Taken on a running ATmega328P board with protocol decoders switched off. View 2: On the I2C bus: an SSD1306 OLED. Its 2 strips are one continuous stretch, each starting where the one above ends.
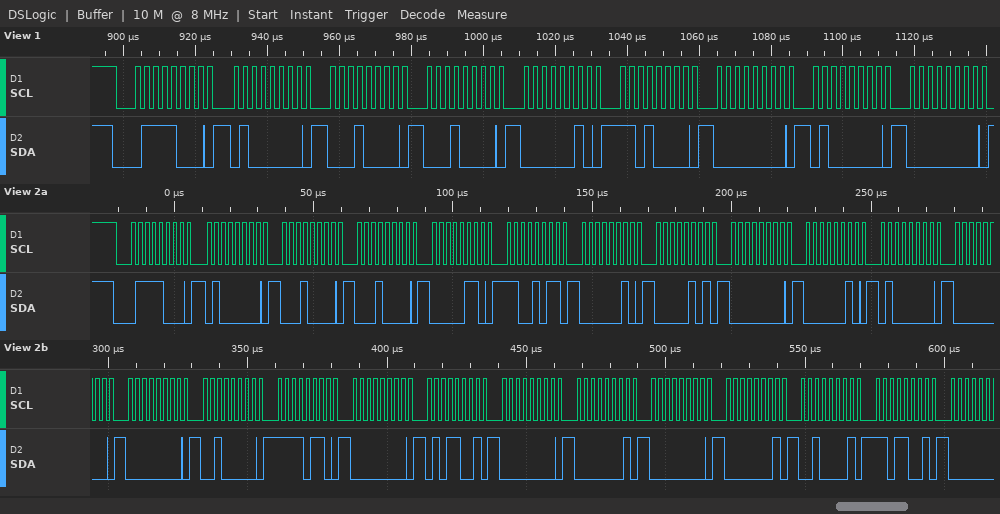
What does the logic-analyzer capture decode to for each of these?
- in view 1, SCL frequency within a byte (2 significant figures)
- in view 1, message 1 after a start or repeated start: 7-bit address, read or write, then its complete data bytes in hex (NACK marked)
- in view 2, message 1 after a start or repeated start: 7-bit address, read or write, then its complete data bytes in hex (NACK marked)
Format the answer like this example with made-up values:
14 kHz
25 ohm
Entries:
400 kHz
0x3C write: 40 10 10 02 D0 00 40 00
0x3C write: 40 10 10 06 CB 02 05 00 02 40 00 00 20 F6 00 59 00 01 00 01 21 D9
